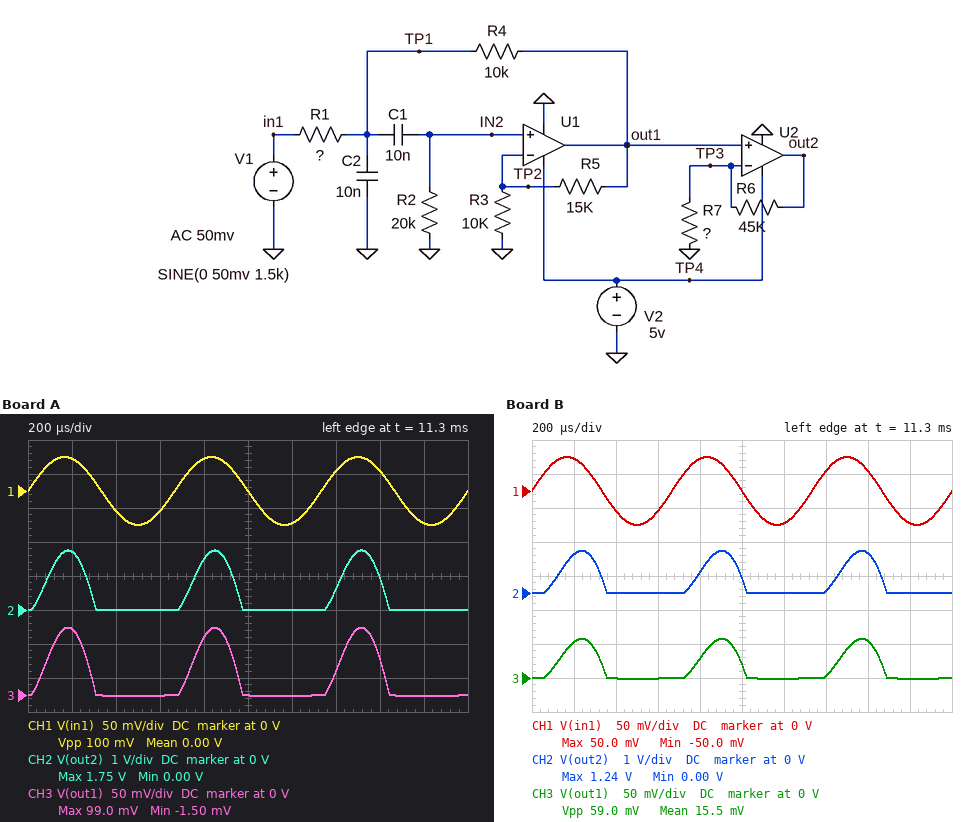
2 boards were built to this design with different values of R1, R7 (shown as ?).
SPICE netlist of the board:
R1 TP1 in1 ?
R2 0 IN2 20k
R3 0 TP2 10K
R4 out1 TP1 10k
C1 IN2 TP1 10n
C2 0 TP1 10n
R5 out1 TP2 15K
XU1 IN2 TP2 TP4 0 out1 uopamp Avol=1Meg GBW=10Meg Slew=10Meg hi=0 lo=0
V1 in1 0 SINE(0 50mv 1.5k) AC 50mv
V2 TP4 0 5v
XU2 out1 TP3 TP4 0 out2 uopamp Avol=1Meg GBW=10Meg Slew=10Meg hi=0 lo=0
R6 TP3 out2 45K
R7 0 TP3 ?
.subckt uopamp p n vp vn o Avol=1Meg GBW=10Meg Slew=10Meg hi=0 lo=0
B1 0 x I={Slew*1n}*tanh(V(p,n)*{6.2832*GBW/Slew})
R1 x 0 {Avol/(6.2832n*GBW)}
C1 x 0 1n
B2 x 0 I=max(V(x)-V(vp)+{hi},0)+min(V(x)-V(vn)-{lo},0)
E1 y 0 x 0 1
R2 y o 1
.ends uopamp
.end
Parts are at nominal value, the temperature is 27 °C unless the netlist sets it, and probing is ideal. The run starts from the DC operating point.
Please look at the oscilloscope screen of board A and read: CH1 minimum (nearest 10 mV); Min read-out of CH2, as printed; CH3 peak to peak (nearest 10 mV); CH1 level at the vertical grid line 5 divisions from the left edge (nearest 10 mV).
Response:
-50 mV
0.00 V
100 mV
0 V
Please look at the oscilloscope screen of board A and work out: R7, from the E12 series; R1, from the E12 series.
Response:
2.7 kΩ
8.2 kΩ
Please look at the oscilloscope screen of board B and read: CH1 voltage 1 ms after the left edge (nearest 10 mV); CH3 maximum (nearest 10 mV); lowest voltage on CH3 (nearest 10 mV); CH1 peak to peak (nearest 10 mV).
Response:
0 V
60 mV
0 V
100 mV
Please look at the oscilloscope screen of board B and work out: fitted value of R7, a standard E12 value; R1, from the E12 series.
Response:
2.2 kΩ
22 kΩ
